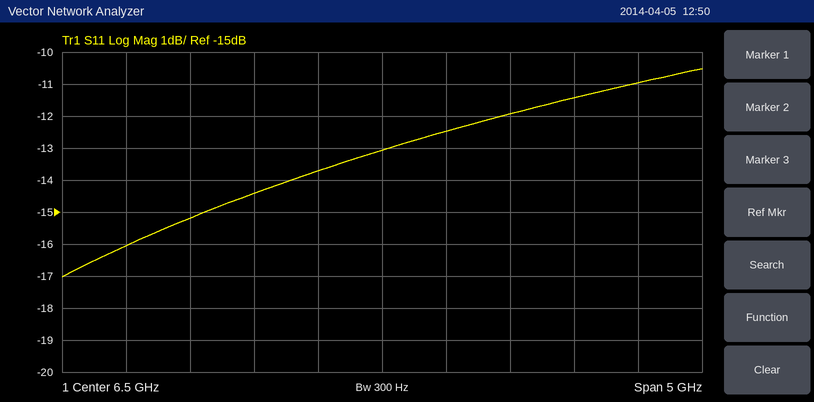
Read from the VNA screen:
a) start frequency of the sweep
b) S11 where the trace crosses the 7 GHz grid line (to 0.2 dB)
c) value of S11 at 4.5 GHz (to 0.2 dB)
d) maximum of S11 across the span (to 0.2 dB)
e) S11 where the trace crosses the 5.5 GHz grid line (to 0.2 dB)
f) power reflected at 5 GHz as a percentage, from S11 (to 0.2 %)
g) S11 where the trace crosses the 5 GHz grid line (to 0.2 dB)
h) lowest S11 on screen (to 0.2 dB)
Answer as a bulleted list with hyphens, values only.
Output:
- 4 GHz
- -12.4 dB
- -16.0 dB
- -10.6 dB
- -14.4 dB
- 3.0 %
- -15.2 dB
- -17.0 dB
